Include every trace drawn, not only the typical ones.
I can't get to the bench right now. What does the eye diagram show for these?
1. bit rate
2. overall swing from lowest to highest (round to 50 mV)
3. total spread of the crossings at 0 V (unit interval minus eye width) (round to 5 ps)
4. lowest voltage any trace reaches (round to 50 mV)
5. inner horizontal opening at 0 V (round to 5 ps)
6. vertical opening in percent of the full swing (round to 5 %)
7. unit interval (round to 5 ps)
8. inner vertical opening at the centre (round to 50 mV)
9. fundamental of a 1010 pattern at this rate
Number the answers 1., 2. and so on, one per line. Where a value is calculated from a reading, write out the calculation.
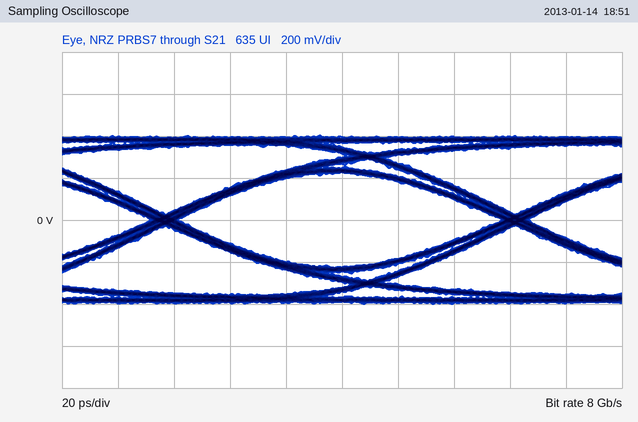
1. 8 Gb/s
2. 800 mV
3. 10 ps
4. -400 mV
5. 115 ps
6. 450 mV / 800 mV ≈ 56.2 %, so 55 % to the nearest 5 %
7. 125 ps
8. 450 mV
9. 4 GHz
